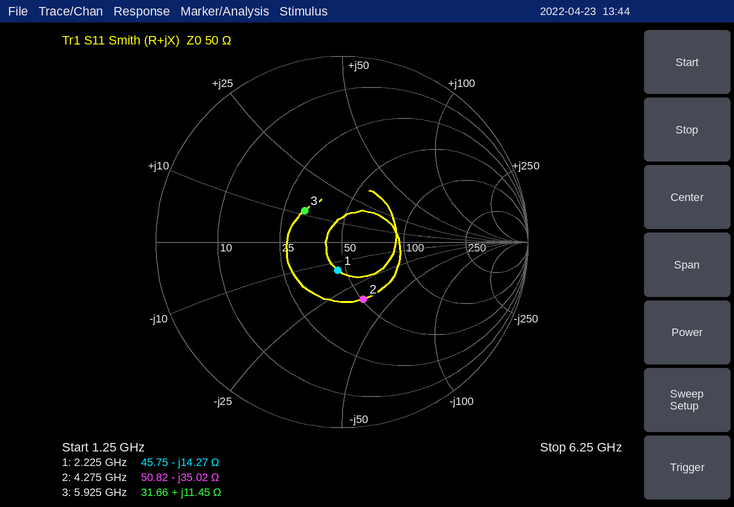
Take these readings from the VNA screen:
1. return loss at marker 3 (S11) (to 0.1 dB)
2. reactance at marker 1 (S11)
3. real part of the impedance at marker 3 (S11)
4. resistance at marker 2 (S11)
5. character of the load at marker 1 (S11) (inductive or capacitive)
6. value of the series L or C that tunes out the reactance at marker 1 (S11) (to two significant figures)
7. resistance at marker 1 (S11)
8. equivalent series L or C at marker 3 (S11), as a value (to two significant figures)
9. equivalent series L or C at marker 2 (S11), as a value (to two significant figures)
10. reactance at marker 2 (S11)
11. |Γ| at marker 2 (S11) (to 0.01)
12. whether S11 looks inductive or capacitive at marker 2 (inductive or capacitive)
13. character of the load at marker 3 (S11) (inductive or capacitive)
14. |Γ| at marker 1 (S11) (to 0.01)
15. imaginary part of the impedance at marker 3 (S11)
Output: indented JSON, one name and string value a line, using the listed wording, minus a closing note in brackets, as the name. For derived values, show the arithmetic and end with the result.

{
  "return loss at marker 3 (S11)": "11.6 dB",
  "reactance at marker 1": "-14.27 Ω",
  "real part of the impedance at marker 3": "31.66 Ω",
  "resistance at marker 2": "50.82 Ω",
  "character of the load at marker 1 (S11)": "capacitive",
  "value of the series L or C that tunes out the reactance at marker 1 (S11)": "L = 14.27 Ω/(2π × 2.225 GHz) ≈ 1.0 nH",
  "resistance at marker 1": "45.75 Ω",
  "equivalent series L or C at marker 3 (S11), as a value": "L = 11.45 Ω/(2π × 5.925 GHz) ≈ 308 pH, so 310 pH to two significant figures",
  "equivalent series L or C at marker 2 (S11), as a value": "C = 1/(2π × 4.275 GHz × 35.02 Ω) ≈ 1.1 pF",
  "reactance at marker 2": "-35.02 Ω",
  "|Γ| at marker 2 (S11)": "0.33",
  "whether S11 looks inductive or capacitive at marker 2": "capacitive",
  "character of the load at marker 3 (S11)": "inductive",
  "|Γ| at marker 1 (S11)": "0.15",
  "imaginary part of the impedance at marker 3": "+11.45 Ω"
}
